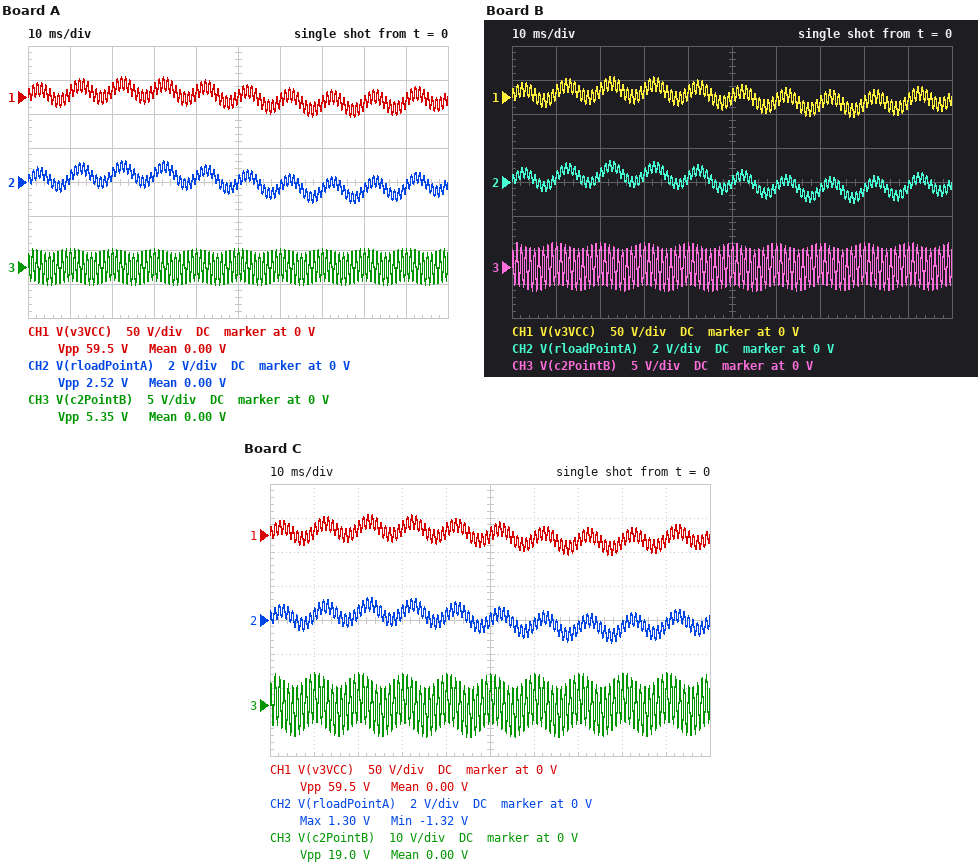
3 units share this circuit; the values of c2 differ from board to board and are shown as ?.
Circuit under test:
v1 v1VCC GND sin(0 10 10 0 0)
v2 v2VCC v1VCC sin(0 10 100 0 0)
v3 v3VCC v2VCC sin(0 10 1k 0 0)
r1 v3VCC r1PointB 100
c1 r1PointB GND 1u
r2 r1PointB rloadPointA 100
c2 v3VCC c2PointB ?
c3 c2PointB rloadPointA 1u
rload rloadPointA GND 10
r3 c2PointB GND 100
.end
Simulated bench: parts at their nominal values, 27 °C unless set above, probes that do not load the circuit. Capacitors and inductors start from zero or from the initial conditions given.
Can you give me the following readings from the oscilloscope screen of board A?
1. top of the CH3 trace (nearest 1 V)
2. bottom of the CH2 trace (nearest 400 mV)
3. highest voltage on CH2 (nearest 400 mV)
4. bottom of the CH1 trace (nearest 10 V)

3 V
-1.2 V
1.2 V
-30 V
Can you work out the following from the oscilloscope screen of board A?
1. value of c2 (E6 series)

470 nF
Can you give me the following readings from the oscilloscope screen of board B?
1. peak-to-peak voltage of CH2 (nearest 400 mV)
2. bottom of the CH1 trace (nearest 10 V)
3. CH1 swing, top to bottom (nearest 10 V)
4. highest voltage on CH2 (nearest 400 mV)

2.4 V
-30 V
60 V
1.2 V
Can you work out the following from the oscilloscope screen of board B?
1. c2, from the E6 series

680 nF
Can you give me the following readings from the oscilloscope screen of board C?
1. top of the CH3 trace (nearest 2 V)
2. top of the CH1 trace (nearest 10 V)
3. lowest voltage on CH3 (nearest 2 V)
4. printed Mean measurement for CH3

10 V
30 V
-10 V
0.00 V
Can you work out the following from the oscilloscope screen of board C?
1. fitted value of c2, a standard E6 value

3.3 µF
